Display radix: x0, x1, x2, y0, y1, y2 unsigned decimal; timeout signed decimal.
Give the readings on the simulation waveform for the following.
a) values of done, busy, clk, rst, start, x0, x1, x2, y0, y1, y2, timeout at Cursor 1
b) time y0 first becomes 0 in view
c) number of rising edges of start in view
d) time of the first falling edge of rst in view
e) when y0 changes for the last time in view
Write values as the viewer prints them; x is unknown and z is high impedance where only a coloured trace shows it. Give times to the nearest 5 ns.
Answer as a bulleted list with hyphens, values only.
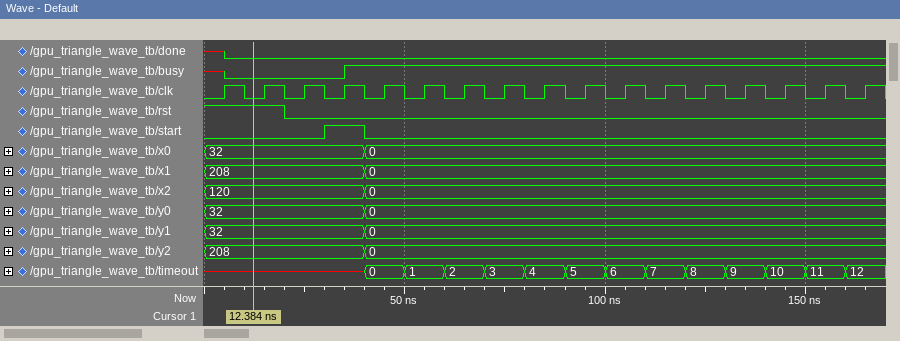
- done=0, busy=0, clk=0, rst=1, start=0, x0=32, x1=208, x2=120, y0=32, y1=32, y2=208, timeout=x
- 40 ns
- 1
- 20 ns
- 40 ns
